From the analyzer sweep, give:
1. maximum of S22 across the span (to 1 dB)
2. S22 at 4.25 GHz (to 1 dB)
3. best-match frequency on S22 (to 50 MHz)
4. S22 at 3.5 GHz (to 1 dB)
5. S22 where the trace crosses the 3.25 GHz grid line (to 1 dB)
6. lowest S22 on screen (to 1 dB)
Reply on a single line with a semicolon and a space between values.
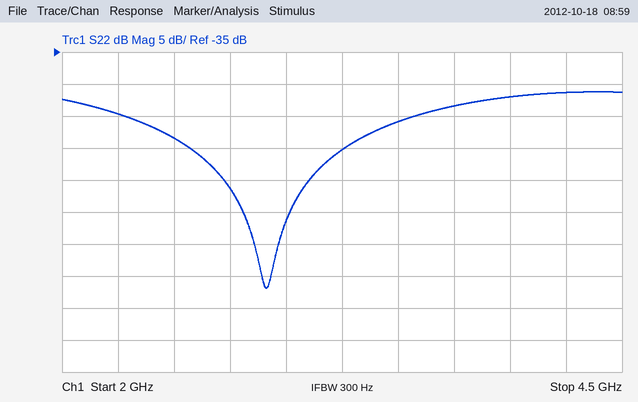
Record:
-41 dB; -41 dB; 2.90 GHz; -46 dB; -50 dB; -72 dB
